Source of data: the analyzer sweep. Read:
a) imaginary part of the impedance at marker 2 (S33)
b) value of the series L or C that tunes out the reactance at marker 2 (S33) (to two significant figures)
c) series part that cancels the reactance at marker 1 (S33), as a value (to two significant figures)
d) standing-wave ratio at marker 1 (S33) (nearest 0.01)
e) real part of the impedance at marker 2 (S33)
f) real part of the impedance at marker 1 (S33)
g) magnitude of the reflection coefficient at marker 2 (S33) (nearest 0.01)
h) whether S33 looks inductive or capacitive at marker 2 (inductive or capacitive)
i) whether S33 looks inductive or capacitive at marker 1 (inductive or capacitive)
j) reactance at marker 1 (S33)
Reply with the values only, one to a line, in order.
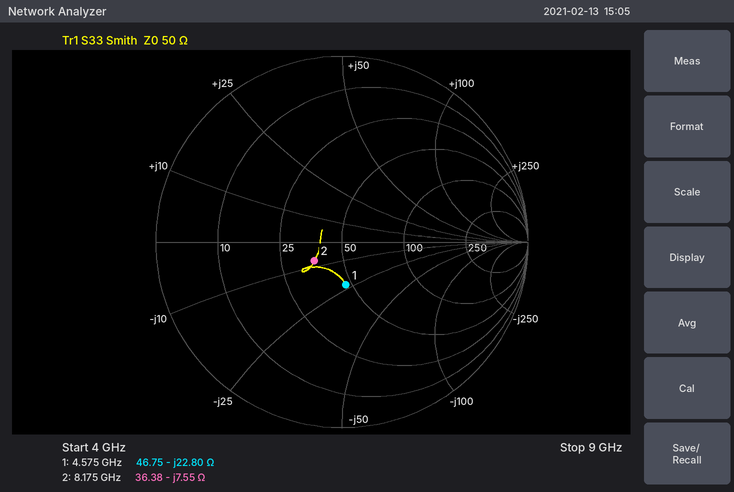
-7.55 Ω
150 pH
790 pH
1.60
36.38 Ω
46.75 Ω
0.18
capacitive
capacitive
-22.80 Ω
